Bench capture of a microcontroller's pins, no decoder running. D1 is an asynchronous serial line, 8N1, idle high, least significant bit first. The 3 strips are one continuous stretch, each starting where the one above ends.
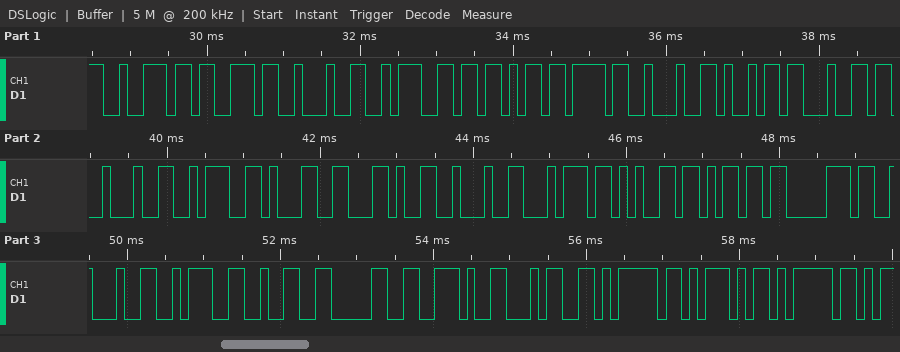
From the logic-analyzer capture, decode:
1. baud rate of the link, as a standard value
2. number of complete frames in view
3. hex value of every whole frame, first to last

9600 baud
27
72 73 22 3A 5B 7B 22 69 64 22 3A 31 2C 22 74 65 6D 70 22 3A 32 30 2E 34 7D 5D 7D
